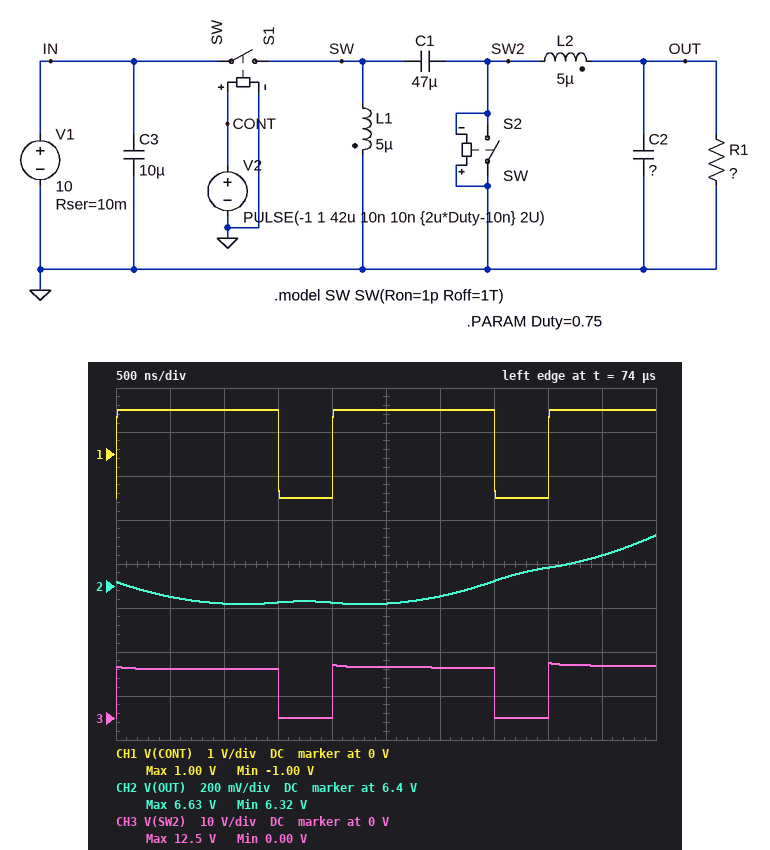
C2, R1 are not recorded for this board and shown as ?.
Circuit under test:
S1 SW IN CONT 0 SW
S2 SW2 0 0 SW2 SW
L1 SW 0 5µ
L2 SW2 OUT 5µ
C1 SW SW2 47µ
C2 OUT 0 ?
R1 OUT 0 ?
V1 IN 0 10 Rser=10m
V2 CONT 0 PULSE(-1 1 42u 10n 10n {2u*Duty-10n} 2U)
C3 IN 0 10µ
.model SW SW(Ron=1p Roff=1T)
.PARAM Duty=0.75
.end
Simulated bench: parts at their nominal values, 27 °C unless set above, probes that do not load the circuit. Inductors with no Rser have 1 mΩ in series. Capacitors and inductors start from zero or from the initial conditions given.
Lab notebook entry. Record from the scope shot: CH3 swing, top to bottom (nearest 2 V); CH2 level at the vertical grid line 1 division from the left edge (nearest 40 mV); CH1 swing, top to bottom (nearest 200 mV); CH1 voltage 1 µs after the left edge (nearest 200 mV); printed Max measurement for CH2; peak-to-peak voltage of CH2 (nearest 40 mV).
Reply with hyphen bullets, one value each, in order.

- 12 V
- 6.36 V
- 2.0 V
- 1.0 V
- 6.63 V
- 320 mV
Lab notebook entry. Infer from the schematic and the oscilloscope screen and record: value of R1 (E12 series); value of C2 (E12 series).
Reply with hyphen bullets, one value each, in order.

- 1.8 Ω
- 6.8 µF
